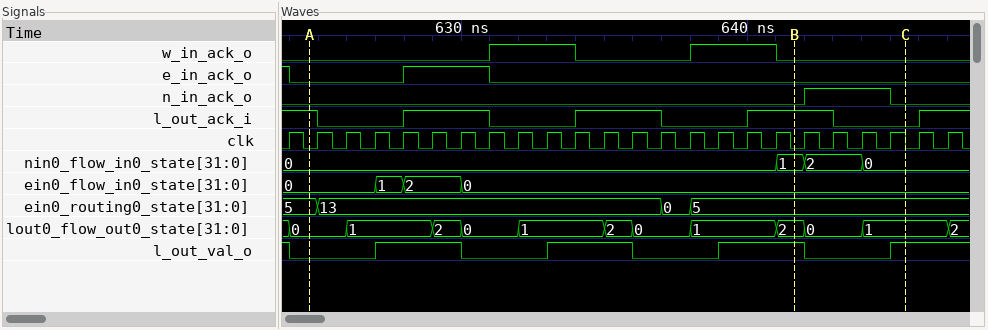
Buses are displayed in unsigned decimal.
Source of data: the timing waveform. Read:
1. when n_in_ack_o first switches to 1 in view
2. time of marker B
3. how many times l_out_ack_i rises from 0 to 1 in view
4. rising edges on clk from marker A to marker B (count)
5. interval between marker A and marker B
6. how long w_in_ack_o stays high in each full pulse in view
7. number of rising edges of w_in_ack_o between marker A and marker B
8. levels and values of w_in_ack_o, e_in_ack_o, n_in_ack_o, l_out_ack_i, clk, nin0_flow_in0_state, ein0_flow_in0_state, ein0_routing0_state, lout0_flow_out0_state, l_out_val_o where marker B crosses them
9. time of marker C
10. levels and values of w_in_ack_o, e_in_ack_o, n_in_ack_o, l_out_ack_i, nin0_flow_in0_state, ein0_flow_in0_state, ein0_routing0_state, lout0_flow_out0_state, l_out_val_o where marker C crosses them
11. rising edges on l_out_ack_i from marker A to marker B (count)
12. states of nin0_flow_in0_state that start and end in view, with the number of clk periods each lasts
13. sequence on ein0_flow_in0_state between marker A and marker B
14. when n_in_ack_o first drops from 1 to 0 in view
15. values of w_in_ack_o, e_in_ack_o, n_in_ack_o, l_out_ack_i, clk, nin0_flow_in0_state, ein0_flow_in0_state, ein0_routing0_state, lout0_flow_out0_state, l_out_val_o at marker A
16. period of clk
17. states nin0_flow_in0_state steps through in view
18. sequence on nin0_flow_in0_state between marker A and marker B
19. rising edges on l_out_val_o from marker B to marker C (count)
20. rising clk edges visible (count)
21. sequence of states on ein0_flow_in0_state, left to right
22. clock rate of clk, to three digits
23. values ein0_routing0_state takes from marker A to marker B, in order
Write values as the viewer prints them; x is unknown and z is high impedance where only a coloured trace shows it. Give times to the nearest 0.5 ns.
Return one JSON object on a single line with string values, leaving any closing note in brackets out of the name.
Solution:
{"when n_in_ack_o first switches to 1 in view": "642 ns", "time of marker B": "641.5 ns", "how many times l_out_ack_i rises from 0 to 1 in view": "4", "rising edges on clk from marker A to marker B": "17", "interval between marker A and marker B": "17 ns", "how long w_in_ack_o stays high in each full pulse in view": "3 ns, 3 ns", "number of rising edges of w_in_ack_o between marker A and marker B": "2", "levels and values of w_in_ack_o, e_in_ack_o, n_in_ack_o, l_out_ack_i, clk, nin0_flow_in0_state, ein0_flow_in0_state, ein0_routing0_state, lout0_flow_out0_state, l_out_val_o where marker B crosses them": "w_in_ack_o=0, e_in_ack_o=0, n_in_ack_o=0, l_out_ack_i=1, clk=0, nin0_flow_in0_state=1, ein0_flow_in0_state=0, ein0_routing0_state=5, lout0_flow_out0_state=2, l_out_val_o=1", "time of marker C": "645.5 ns", "levels and values of w_in_ack_o, e_in_ack_o, n_in_ack_o, l_out_ack_i, nin0_flow_in0_state, ein0_flow_in0_state, ein0_routing0_state, lout0_flow_out0_state, l_out_val_o where marker C crosses them": "w_in_ack_o=0, e_in_ack_o=0, n_in_ack_o=0, l_out_ack_i=0, nin0_flow_in0_state=0, ein0_flow_in0_state=0, ein0_routing0_state=5, lout0_flow_out0_state=1, l_out_val_o=1", "rising edges on l_out_ack_i from marker A to marker B": "3", "states of nin0_flow_in0_state that start and end in view, with the number of clk periods each lasts": "1: 1, 2: 2", "sequence on ein0_flow_in0_state between marker A and marker B": "0, 1, 2, 0", "when n_in_ack_o first drops from 1 to 0 in view": "645 ns", "values of w_in_ack_o, e_in_ack_o, n_in_ack_o, l_out_ack_i, clk, nin0_flow_in0_state, ein0_flow_in0_state, ein0_routing0_state, lout0_flow_out0_state, l_out_val_o at marker A": "w_in_ack_o=0, e_in_ack_o=0, n_in_ack_o=0, l_out_ack_i=1, clk=0, nin0_flow_in0_state=0, ein0_flow_in0_state=0, ein0_routing0_state=5, lout0_flow_out0_state=0, l_out_val_o=0", "period of clk": "1 ns", "states nin0_flow_in0_state steps through in view": "0, 1, 2, 0", "sequence on nin0_flow_in0_state between marker A and marker B": "0, 1", "rising edges on l_out_val_o from marker B to marker C": "1", "rising clk edges visible": "24", "sequence of states on ein0_flow_in0_state, left to right": "0, 1, 2, 0", "clock rate of clk, to three digits": "1.00 GHz", "values ein0_routing0_state takes from marker A to marker B, in order": "5, 13, 0, 5"}
